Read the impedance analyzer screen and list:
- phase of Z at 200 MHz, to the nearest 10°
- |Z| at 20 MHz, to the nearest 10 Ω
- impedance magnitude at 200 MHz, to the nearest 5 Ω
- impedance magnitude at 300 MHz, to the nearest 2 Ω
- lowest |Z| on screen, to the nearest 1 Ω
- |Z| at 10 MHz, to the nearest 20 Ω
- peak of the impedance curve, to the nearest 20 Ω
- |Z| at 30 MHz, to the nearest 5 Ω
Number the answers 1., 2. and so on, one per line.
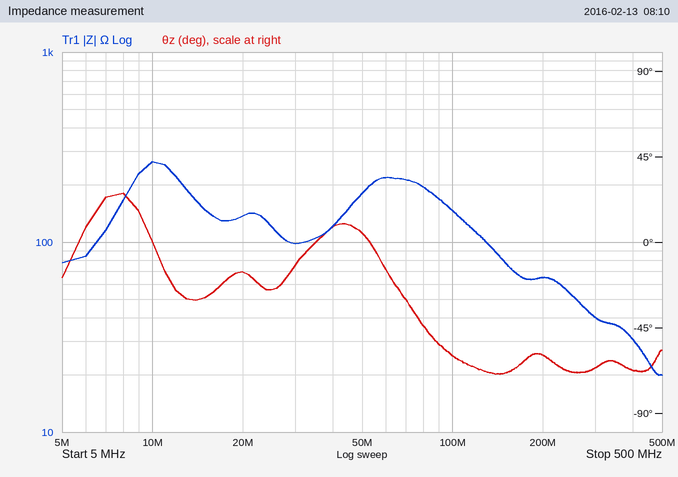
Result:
1. -60°
2. 140 Ω
3. 65 Ω
4. 40 Ω
5. 20 Ω
6. 260 Ω
7. 260 Ω
8. 100 Ω
